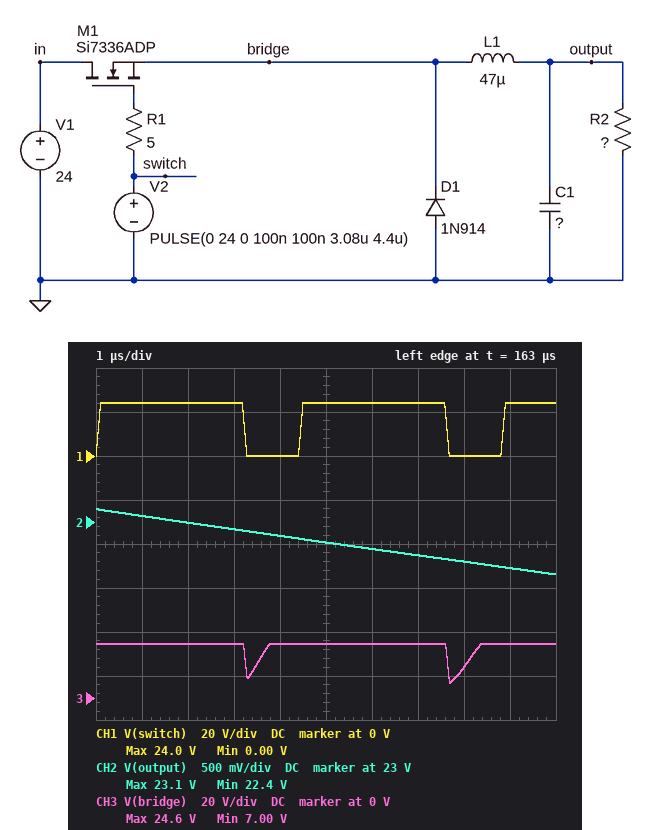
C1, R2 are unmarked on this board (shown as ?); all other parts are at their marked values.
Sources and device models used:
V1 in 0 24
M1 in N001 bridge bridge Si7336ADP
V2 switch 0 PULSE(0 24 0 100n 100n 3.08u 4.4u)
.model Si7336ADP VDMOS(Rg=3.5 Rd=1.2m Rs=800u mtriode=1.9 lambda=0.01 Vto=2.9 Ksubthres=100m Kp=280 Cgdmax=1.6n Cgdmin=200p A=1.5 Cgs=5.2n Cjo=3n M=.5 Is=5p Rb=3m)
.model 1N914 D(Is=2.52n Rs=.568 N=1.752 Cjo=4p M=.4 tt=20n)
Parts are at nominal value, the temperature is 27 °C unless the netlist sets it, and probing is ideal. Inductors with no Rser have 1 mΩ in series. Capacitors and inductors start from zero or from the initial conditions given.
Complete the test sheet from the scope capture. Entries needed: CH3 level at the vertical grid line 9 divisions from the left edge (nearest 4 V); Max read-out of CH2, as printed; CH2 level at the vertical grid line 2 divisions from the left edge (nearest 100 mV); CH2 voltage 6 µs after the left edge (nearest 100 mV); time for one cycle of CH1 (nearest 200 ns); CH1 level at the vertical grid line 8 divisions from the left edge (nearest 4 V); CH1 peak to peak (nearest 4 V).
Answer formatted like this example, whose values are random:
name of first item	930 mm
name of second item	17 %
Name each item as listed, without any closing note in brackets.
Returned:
CH3 level at the vertical grid line 9 divisions from the left edge	24 V
Max read-out of CH2, as printed	23.1 V
CH2 level at the vertical grid line 2 divisions from the left edge	23.0 V
CH2 voltage 6 µs after the left edge	22.7 V
time for one cycle of CH1	4.4 µs
CH1 level at the vertical grid line 8 divisions from the left edge	0 V
CH1 peak to peak	24 V
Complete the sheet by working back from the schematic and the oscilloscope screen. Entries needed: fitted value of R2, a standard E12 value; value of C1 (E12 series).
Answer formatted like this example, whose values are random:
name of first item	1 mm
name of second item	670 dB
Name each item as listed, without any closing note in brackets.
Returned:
fitted value of R2, a standard E12 value	10 Ω
value of C1	33 µF
